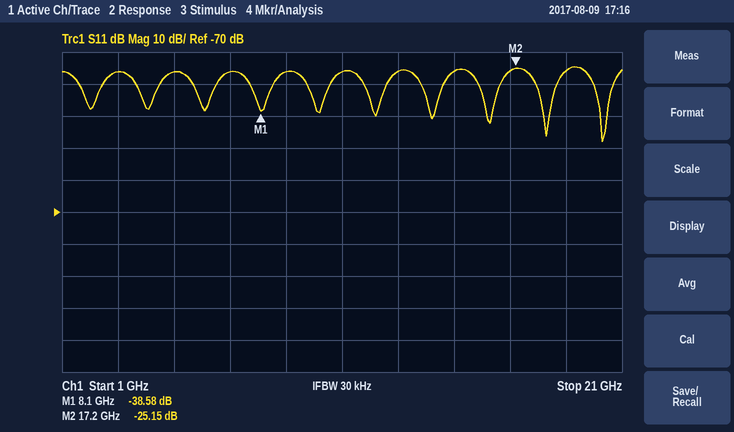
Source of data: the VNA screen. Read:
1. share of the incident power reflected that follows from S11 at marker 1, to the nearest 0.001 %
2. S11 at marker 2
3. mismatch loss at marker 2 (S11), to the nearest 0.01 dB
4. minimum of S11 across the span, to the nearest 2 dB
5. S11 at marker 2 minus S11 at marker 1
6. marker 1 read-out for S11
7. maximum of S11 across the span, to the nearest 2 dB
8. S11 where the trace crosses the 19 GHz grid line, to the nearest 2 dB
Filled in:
0.014 %
-25.15 dB
0.01 dB
-48 dB
13.43 dB
-38.58 dB
-24 dB
-26 dB
